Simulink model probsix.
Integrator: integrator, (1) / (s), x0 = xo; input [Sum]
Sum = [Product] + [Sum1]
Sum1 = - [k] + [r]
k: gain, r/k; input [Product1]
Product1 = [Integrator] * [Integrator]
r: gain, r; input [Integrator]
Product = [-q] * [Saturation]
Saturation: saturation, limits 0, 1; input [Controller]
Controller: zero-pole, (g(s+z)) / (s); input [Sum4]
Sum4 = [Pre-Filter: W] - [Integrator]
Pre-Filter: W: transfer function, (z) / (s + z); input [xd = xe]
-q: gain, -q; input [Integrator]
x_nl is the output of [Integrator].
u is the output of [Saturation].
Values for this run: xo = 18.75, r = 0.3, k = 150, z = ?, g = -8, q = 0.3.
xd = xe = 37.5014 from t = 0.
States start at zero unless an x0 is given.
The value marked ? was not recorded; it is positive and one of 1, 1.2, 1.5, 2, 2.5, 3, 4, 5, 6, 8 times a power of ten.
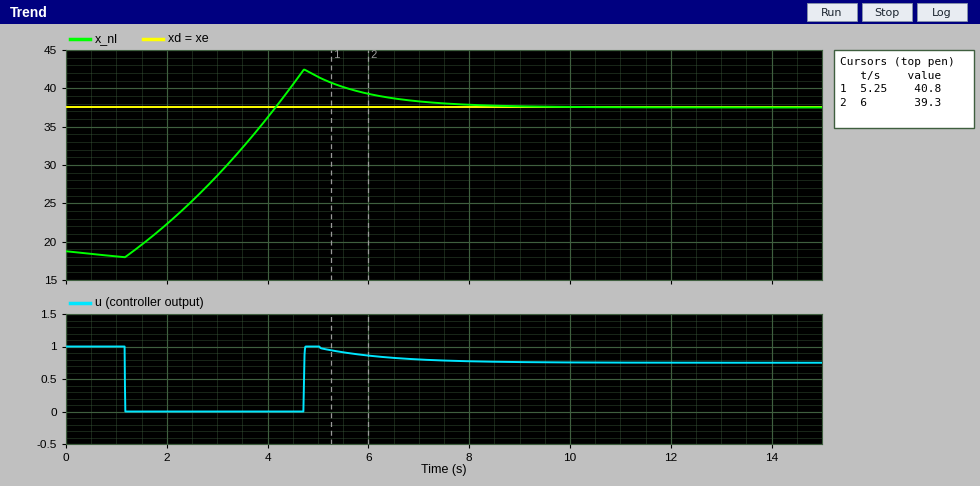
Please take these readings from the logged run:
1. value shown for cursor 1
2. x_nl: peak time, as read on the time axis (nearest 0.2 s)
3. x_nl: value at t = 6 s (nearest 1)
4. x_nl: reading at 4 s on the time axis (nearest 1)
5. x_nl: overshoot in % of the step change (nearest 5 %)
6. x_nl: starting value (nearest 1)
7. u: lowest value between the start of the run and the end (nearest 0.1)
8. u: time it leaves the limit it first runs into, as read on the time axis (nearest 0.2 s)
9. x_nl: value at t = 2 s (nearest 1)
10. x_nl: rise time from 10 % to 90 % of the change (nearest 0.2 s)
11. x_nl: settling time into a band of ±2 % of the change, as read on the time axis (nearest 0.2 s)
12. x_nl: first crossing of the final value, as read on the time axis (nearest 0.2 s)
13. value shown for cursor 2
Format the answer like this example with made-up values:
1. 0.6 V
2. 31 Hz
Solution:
1. 40.8
2. 4.8 s
3. 39
4. 36
5. 25 %
6. 19
7. 0.0
8. 1.2 s
9. 22
10. 2.2 s
11. 8.0 s
12. 4.2 s
13. 39.3
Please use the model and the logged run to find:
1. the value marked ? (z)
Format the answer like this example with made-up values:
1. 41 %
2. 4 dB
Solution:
1. 0.8
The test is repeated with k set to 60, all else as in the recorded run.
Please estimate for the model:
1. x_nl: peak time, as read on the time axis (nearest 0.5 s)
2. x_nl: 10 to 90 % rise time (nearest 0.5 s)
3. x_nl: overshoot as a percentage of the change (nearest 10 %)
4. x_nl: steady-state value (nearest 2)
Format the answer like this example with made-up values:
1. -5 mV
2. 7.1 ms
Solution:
1. 8.5 s
2. 3.5 s
3. 50 %
4. 38
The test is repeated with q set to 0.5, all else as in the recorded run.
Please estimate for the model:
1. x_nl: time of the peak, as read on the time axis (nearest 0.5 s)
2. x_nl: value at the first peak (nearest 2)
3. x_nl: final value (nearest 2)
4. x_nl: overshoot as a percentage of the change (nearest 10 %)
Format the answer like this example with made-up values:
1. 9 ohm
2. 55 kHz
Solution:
1. 5.5 s
2. 48
3. 38
4. 50 %
